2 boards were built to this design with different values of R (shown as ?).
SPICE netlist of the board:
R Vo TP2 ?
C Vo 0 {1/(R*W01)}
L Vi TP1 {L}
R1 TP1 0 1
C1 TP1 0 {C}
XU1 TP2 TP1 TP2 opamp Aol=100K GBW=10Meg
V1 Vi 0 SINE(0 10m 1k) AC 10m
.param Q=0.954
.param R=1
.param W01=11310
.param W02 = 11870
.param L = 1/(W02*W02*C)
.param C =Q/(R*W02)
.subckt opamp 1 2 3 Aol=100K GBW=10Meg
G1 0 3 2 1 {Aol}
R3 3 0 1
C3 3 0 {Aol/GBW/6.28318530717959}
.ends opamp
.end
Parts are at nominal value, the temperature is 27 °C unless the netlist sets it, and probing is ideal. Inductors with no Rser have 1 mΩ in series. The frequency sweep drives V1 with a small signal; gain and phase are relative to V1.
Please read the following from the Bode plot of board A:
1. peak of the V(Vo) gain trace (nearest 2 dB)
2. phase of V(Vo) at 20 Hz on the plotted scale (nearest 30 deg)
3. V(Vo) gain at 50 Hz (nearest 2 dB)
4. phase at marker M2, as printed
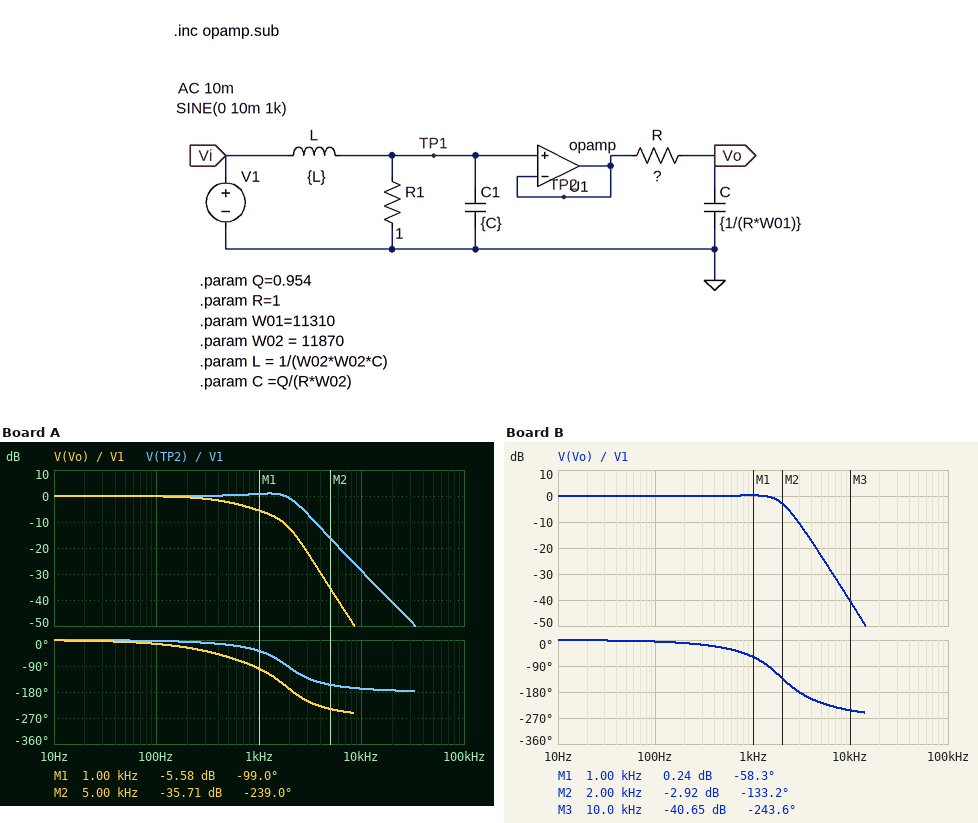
0 dB
0 deg
0 dB
-239.0 deg
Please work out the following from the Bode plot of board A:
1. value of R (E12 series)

3.3 Ω
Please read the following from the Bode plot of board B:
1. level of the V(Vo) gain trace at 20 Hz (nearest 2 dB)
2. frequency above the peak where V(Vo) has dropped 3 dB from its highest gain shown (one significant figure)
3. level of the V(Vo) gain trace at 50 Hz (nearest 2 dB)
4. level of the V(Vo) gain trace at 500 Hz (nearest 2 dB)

0 dB
2 kHz
0 dB
0 dB
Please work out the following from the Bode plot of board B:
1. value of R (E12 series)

0.68 Ω
